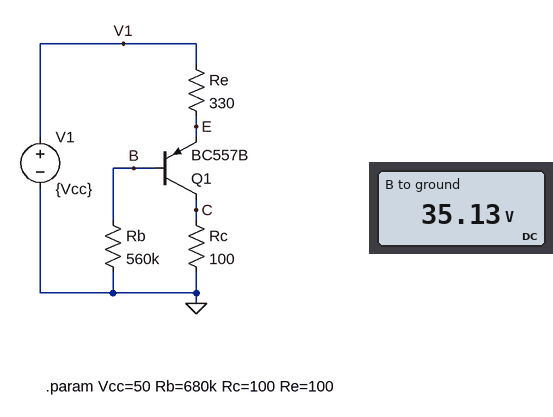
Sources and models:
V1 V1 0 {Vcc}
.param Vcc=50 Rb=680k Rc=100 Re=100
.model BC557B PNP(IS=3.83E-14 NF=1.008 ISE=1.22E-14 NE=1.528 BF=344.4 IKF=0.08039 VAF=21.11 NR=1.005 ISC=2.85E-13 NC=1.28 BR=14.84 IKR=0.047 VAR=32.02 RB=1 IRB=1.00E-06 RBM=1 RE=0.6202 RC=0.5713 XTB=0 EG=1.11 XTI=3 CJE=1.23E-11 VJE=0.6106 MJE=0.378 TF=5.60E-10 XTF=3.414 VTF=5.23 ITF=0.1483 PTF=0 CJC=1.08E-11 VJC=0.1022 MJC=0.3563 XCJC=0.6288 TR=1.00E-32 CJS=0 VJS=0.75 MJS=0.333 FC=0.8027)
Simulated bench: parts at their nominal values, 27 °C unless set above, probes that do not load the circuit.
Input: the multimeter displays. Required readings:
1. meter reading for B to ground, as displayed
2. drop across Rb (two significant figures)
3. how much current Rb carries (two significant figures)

35.13 V
35 V
63 µA
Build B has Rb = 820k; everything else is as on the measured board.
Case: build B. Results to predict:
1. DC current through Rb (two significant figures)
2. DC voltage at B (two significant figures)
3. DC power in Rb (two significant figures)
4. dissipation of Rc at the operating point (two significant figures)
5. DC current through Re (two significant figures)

46 µA
38 V
1.7 mW
120 mW
35 mA
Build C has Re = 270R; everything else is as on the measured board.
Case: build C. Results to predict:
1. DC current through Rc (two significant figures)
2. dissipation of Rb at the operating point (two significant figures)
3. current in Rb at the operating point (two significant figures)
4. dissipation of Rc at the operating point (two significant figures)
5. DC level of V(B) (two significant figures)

46 mA
2.4 mW
66 µA
210 mW
37 V
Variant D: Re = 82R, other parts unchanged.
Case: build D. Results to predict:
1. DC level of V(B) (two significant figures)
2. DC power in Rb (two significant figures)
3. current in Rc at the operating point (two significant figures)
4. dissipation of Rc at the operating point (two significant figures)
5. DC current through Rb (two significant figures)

44 V
3.5 mW
60 mA
360 mW
79 µA
